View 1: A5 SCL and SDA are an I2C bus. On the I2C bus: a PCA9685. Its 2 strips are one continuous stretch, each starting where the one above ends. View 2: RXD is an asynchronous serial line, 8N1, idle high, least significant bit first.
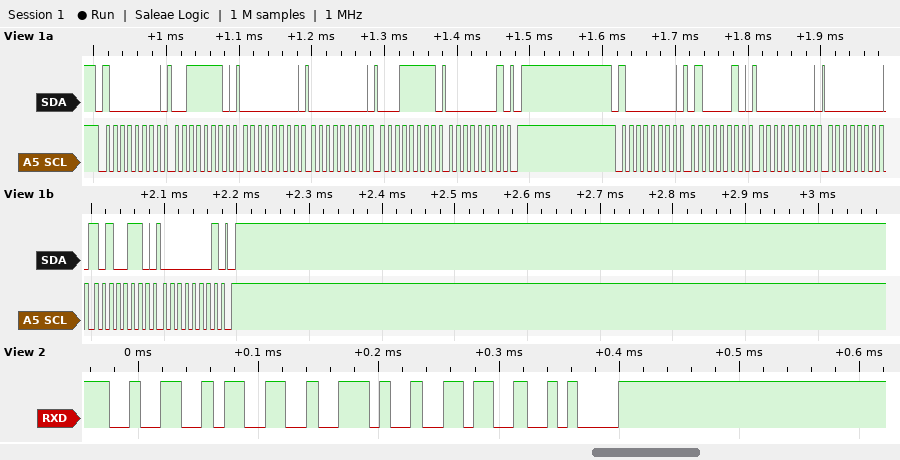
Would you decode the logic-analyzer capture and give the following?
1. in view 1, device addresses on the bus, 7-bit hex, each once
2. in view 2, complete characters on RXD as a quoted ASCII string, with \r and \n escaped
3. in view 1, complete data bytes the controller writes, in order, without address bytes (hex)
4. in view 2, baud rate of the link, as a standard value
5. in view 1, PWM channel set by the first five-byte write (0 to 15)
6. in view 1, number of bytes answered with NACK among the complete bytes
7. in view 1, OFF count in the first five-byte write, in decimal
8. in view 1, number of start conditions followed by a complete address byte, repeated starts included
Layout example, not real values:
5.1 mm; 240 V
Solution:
0x40; "23.6\n"; 3E 00 00 1F 01 42 00 00 A6 01; 115200 baud; 14; 0; 287; 2
